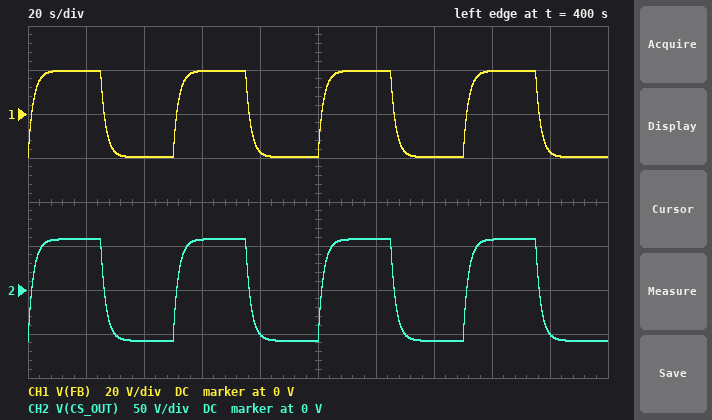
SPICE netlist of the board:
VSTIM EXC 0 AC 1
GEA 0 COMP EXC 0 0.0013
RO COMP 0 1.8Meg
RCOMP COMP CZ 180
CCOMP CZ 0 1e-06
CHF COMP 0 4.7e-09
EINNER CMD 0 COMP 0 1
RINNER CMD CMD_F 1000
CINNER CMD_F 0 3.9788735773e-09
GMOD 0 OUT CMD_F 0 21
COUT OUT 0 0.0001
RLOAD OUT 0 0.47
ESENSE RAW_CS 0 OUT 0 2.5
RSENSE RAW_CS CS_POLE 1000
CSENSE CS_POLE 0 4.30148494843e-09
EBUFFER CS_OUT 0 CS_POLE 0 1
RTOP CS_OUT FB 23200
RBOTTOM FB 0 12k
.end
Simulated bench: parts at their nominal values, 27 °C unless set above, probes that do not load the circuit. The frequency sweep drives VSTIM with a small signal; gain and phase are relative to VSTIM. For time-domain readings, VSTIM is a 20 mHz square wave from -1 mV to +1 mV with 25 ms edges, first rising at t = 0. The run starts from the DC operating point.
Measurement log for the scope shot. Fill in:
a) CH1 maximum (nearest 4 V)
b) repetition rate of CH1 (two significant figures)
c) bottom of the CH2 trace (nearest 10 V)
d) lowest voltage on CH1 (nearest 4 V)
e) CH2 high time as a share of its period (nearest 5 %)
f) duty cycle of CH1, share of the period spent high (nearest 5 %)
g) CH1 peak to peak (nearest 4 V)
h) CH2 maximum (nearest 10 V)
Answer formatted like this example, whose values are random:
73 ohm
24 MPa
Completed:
20 V
20 mHz
-60 V
-20 V
50 %
50 %
40 V
60 V
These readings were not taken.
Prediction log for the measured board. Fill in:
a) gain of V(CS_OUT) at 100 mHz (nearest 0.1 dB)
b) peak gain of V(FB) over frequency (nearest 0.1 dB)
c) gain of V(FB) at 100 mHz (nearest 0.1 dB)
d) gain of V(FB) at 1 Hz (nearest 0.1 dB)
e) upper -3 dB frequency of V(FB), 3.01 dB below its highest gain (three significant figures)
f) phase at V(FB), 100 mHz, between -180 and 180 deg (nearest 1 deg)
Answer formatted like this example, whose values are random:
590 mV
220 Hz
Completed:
91.6 dB
85.9 dB
82.3 dB
64.7 dB
88.0 mHz
-49 deg
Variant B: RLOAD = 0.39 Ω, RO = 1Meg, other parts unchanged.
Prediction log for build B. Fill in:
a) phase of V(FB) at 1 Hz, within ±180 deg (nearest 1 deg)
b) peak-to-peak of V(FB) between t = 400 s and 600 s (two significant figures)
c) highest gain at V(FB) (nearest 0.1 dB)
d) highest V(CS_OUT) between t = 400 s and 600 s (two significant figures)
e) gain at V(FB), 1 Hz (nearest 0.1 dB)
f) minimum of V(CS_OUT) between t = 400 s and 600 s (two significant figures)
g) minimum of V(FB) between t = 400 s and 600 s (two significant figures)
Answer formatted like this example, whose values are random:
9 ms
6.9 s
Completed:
-81 deg
18 V
79.2 dB
27 V
63.0 dB
-27 V
-9.1 V
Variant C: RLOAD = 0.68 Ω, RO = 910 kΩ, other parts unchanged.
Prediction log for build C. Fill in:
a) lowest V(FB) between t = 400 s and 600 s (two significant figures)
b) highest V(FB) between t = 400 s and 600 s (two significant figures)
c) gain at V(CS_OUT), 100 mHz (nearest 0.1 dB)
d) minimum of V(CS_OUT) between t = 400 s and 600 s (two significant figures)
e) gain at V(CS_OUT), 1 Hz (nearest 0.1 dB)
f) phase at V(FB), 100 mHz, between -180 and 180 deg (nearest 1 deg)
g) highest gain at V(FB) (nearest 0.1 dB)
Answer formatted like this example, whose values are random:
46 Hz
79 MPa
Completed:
-14 V
14 V
91.3 dB
-42 V
77.2 dB
-30 deg
83.2 dB
